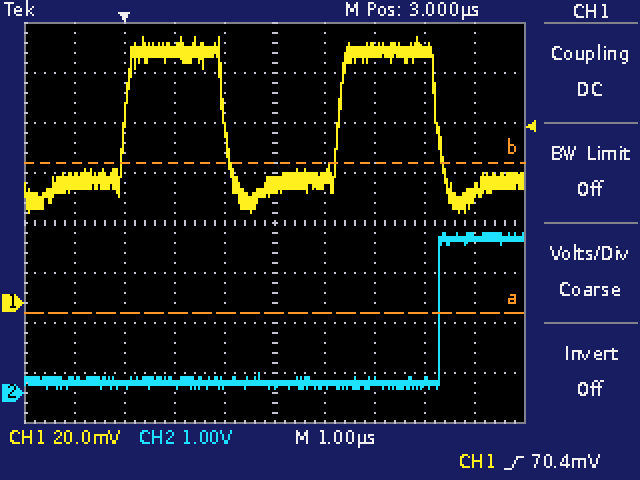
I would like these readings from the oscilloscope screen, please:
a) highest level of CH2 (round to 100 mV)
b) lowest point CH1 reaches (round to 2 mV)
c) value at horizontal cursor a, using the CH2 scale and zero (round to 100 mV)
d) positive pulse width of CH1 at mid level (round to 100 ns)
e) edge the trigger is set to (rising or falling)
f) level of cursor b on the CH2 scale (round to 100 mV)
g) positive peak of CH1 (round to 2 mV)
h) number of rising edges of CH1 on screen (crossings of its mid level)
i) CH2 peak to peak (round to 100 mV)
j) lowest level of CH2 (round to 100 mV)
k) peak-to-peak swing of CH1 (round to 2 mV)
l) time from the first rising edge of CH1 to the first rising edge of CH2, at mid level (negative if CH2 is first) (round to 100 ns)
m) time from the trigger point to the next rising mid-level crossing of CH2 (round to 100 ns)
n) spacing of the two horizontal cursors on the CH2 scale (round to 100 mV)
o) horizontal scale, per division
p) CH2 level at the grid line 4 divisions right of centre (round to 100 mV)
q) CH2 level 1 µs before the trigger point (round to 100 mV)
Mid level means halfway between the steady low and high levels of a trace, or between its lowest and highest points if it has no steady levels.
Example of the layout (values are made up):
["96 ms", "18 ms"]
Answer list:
["3.2 V", "36 mV", "1.6 V", "2.0 µs", "rising", "4.6 V", "106 mV", "2", "3.1 V", "100 mV", "70 mV", "+6.3 µs", "6.3 µs", "3.0 V", "1 µs", "3.1 V", "200 mV"]
